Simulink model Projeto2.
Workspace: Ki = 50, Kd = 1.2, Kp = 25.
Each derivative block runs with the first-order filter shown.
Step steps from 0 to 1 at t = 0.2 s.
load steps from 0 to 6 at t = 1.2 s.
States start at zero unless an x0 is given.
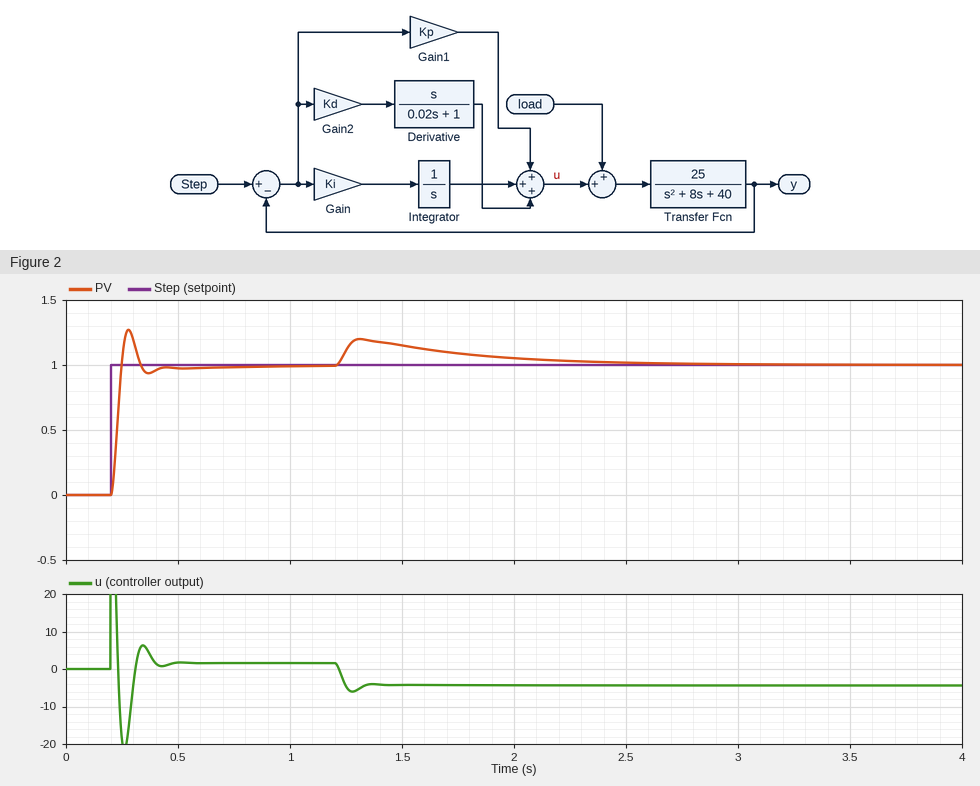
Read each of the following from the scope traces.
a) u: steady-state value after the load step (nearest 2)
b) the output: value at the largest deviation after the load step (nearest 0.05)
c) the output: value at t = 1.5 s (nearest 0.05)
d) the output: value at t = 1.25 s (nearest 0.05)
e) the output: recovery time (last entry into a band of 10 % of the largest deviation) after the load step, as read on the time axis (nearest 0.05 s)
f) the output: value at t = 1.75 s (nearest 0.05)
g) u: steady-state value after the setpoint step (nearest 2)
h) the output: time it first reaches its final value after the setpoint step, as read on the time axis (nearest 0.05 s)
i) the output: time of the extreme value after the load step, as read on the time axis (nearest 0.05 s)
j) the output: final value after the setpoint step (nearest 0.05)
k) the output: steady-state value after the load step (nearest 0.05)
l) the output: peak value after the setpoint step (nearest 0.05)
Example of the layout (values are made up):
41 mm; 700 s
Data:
-4; 1.20; 1.15; 1.10; 2.45 s; 1.10; 2; 0.25 s; 1.30 s; 1.00; 1.00; 1.25
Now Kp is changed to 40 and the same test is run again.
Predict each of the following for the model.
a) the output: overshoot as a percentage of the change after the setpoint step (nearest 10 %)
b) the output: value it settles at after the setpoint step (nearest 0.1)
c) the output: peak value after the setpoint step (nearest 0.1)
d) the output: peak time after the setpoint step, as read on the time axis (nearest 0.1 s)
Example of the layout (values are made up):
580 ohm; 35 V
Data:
40 %; 1.0; 1.4; 0.3 s
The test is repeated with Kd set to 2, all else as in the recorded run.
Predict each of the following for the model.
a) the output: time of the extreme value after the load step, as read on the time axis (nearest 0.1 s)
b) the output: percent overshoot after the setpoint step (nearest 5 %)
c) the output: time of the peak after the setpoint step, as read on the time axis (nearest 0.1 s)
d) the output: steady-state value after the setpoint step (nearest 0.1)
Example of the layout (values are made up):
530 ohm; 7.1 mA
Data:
1.4 s; 25 %; 0.3 s; 1.0
